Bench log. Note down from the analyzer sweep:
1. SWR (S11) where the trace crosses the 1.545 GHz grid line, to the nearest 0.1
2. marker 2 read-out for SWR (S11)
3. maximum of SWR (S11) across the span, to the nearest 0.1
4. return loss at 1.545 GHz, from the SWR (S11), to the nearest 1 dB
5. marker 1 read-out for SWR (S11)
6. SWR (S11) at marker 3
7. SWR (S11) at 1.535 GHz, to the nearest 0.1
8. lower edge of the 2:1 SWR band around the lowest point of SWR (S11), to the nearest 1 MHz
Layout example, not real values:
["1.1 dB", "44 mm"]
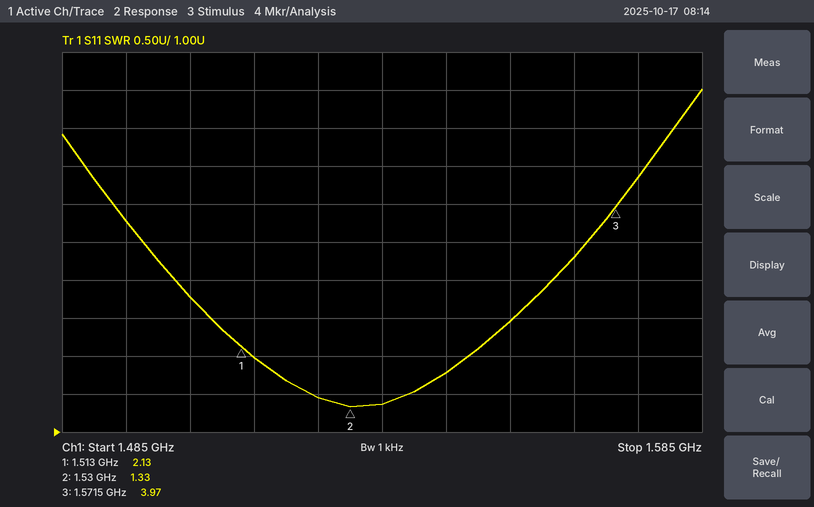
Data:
["1.8", "1.33", "5.5", "11 dB", "2.13", "3.97", "1.4", "1.515 GHz"]
